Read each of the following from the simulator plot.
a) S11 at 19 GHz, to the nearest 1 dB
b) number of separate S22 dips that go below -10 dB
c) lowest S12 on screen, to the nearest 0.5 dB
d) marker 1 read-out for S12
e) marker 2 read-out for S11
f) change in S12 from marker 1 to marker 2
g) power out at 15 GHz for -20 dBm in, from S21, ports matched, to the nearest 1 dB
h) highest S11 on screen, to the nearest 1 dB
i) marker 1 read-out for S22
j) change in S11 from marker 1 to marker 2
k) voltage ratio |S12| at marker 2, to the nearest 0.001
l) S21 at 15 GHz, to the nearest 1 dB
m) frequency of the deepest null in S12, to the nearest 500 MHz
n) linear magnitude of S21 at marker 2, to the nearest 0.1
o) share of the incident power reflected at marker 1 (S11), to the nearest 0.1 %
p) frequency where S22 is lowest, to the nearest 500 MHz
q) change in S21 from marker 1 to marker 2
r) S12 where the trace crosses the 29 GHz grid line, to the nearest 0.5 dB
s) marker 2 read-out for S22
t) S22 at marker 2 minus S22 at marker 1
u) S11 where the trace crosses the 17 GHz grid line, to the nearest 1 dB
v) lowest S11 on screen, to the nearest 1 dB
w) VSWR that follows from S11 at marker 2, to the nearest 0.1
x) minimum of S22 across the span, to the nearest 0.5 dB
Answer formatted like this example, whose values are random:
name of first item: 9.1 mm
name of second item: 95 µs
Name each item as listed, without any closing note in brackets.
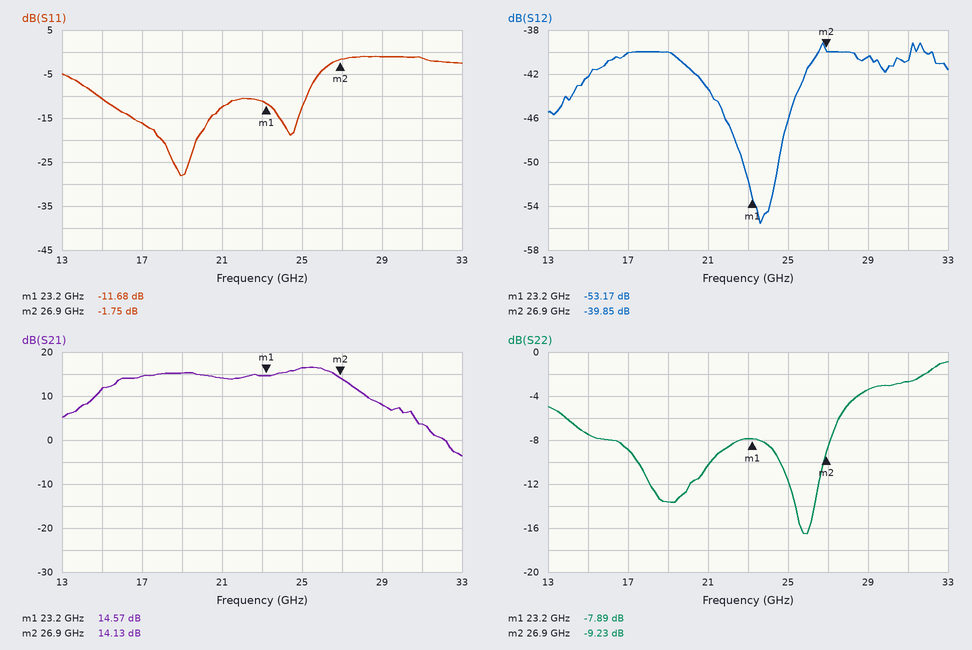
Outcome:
S11 at 19 GHz, to the nearest 1 dB: -28 dB
number of separate S22 dips that go below -10 dB: 2
lowest S12 on screen, to the nearest 0.5 dB: -55.5 dB
marker 1 read-out for S12: -53.17 dB
marker 2 read-out for S11: -1.75 dB
change in S12 from marker 1 to marker 2: 13.32 dB
power out at 15 GHz for -20 dBm in, from S21, ports matched, to the nearest 1 dB: -8 dBm
highest S11 on screen, to the nearest 1 dB: -1 dB
marker 1 read-out for S22: -7.89 dB
change in S11 from marker 1 to marker 2: 9.93 dB
voltage ratio |S12| at marker 2, to the nearest 0.001: 0.010
S21 at 15 GHz, to the nearest 1 dB: 12 dB
frequency of the deepest null in S12, to the nearest 500 MHz: 23.5 GHz
linear magnitude of S21 at marker 2, to the nearest 0.1: 5.1
share of the incident power reflected at marker 1 (S11), to the nearest 0.1 %: 6.8 %
frequency where S22 is lowest, to the nearest 500 MHz: 26.0 GHz
change in S21 from marker 1 to marker 2: -0.44 dB
S12 where the trace crosses the 29 GHz grid line, to the nearest 0.5 dB: -40.5 dB
marker 2 read-out for S22: -9.23 dB
S22 at marker 2 minus S22 at marker 1: -1.34 dB
S11 where the trace crosses the 17 GHz grid line, to the nearest 1 dB: -16 dB
lowest S11 on screen, to the nearest 1 dB: -28 dB
VSWR that follows from S11 at marker 2, to the nearest 0.1: 10.0
minimum of S22 across the span, to the nearest 0.5 dB: -16.5 dB
